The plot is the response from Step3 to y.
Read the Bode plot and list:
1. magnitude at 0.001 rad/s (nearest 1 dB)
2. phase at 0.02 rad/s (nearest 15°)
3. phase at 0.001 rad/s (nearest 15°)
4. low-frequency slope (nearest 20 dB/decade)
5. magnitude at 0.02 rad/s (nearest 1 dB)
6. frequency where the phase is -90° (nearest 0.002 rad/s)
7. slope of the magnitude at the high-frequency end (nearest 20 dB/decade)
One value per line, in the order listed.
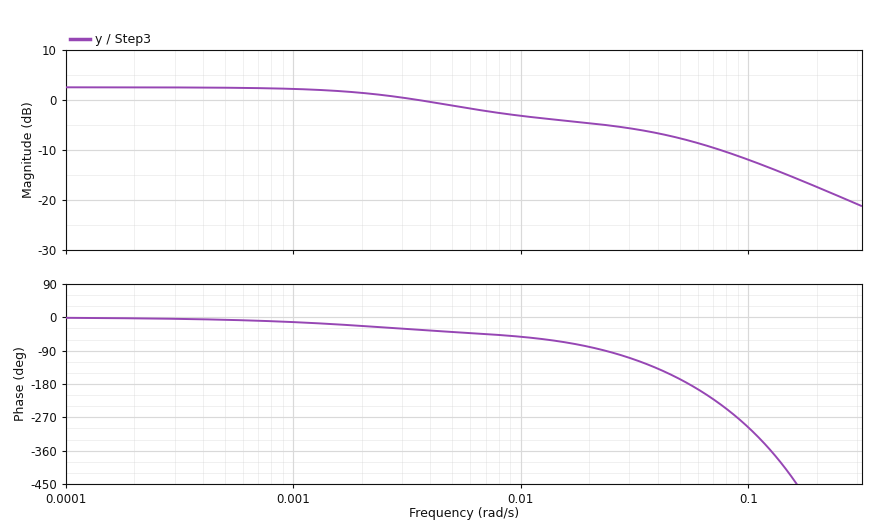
2 dB
-75°
-15°
0 dB/decade
-5 dB
0.024 rad/s
-20 dB/decade
